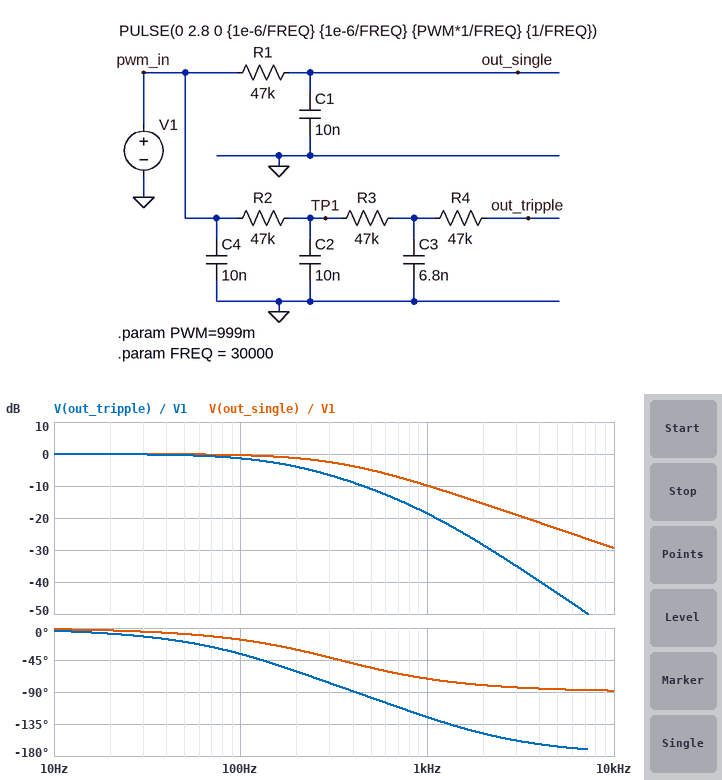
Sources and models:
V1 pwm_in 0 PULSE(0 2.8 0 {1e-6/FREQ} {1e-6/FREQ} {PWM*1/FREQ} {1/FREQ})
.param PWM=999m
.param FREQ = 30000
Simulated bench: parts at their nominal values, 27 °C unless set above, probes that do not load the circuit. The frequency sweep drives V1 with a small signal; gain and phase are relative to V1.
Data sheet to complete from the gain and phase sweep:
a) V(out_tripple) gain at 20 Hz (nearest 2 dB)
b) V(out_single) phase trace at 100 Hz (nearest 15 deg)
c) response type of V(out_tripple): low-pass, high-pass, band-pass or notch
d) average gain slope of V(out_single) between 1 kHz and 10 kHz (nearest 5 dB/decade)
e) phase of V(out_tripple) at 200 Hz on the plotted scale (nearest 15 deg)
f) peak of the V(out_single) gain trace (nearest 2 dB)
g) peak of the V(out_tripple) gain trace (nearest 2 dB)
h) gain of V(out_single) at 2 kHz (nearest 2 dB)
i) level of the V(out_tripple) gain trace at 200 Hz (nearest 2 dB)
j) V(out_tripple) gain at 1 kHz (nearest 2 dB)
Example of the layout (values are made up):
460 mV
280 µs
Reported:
0 dB
-15 deg
low-pass
-20 dB/decade
-60 deg
0 dB
0 dB
-16 dB
-4 dB
-18 dB
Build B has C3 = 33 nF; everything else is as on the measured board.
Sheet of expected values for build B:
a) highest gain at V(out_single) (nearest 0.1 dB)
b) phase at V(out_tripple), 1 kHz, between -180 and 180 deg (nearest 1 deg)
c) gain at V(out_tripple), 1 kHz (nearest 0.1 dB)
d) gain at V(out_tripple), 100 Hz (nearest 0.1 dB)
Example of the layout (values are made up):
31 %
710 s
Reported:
0 dB
-141 deg
-31.1 dB
-7.4 dB
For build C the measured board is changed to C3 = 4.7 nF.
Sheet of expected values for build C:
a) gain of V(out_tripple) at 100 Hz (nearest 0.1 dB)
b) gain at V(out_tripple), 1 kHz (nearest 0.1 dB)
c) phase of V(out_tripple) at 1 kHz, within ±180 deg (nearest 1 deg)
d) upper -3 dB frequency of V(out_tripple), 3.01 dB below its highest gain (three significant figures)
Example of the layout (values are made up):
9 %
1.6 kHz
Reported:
-1.0 dB
-16.3 dB
-118 deg
199 Hz
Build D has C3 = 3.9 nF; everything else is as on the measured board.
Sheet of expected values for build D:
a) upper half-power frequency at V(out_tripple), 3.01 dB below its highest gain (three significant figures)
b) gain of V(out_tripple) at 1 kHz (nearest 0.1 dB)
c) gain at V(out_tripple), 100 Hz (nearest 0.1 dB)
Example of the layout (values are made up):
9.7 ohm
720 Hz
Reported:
216 Hz
-15.2 dB
-0.8 dB
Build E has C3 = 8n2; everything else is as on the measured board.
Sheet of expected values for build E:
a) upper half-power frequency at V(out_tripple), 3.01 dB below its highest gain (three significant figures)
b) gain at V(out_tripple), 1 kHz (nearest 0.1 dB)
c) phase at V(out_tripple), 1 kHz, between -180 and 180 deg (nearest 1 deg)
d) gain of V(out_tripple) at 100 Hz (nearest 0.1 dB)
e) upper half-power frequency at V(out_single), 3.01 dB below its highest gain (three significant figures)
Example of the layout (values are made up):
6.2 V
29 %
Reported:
145 Hz
-19.9 dB
-128 deg
-1.7 dB
339 Hz
